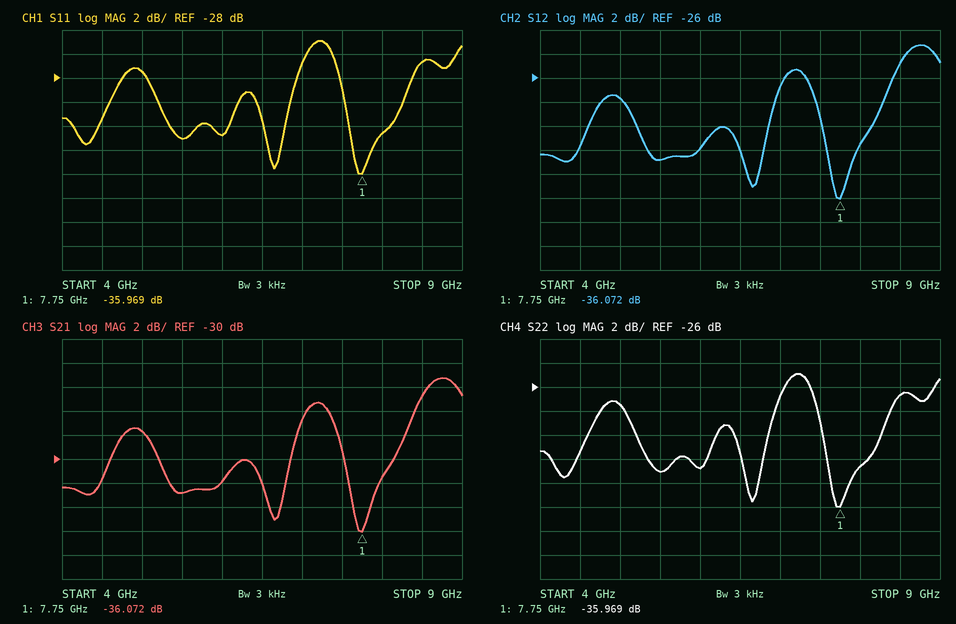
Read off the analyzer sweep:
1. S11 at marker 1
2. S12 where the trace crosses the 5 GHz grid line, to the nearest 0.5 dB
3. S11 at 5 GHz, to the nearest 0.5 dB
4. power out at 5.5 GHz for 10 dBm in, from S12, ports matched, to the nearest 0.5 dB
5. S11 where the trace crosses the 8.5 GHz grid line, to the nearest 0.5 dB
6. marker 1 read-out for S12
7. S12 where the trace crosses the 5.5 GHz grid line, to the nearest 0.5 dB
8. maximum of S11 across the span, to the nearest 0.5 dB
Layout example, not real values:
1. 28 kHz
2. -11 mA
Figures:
1. -35.969 dB
2. -27.5 dB
3. -27.5 dB
4. -23.0 dBm
5. -26.5 dB
6. -36.072 dB
7. -33.0 dB
8. -25.0 dB
